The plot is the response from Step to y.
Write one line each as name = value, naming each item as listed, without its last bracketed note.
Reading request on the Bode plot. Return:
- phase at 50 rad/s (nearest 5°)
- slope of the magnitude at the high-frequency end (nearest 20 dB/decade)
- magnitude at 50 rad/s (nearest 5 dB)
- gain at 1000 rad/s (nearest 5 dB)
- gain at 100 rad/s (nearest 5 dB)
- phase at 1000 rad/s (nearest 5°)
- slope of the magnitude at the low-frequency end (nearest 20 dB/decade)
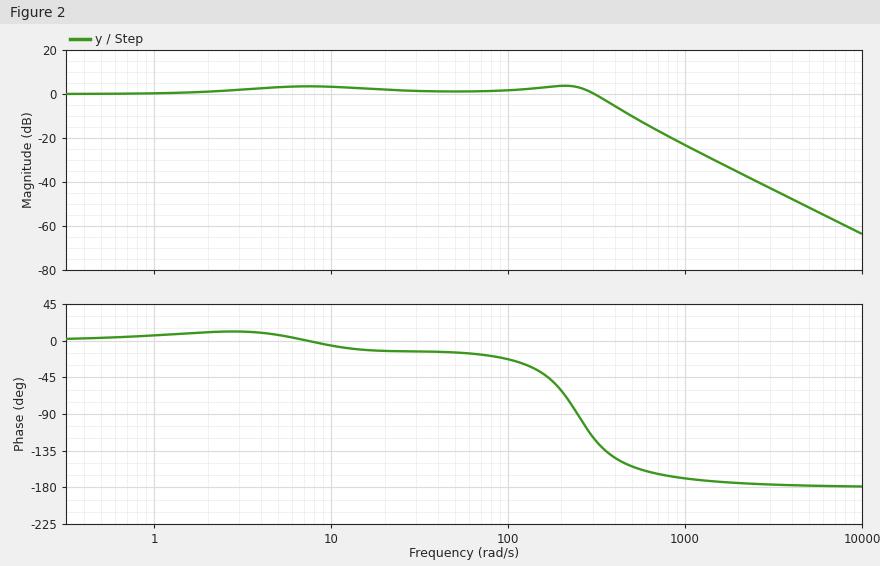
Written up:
phase at 50 rad/s = -15°
slope of the magnitude at the high-frequency end = -40 dB/decade
magnitude at 50 rad/s = 0 dB
gain at 1000 rad/s = -25 dB
gain at 100 rad/s = 0 dB
phase at 1000 rad/s = -170°
slope of the magnitude at the low-frequency end = 0 dB/decade
